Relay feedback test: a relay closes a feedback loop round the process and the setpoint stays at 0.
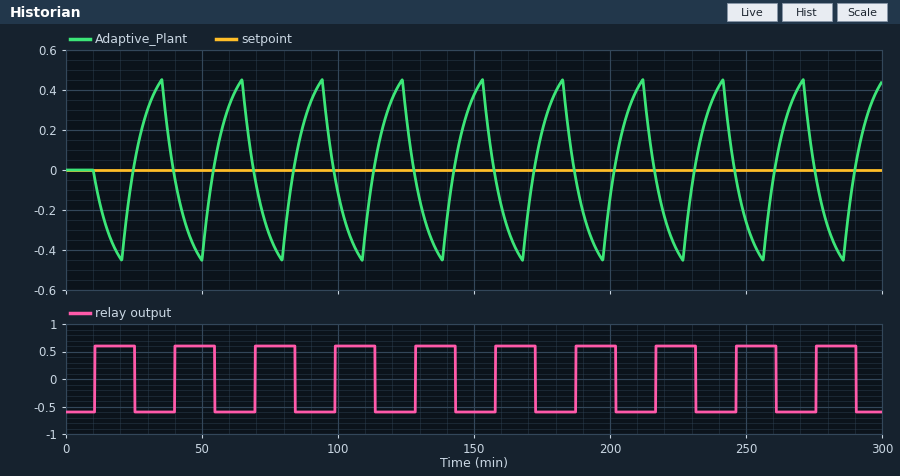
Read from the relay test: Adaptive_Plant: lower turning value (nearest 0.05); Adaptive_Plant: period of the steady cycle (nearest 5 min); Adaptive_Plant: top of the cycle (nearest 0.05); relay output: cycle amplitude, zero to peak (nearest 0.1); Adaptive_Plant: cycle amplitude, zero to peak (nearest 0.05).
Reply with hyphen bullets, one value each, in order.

- -0.45
- 30 min
- 0.45
- 0.6
- 0.45
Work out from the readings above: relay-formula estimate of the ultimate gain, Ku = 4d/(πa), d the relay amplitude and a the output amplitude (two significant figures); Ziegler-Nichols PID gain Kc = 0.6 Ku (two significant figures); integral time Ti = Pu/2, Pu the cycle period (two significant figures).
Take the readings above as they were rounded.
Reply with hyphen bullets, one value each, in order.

- 1.7
- 1.0
- 15 min
